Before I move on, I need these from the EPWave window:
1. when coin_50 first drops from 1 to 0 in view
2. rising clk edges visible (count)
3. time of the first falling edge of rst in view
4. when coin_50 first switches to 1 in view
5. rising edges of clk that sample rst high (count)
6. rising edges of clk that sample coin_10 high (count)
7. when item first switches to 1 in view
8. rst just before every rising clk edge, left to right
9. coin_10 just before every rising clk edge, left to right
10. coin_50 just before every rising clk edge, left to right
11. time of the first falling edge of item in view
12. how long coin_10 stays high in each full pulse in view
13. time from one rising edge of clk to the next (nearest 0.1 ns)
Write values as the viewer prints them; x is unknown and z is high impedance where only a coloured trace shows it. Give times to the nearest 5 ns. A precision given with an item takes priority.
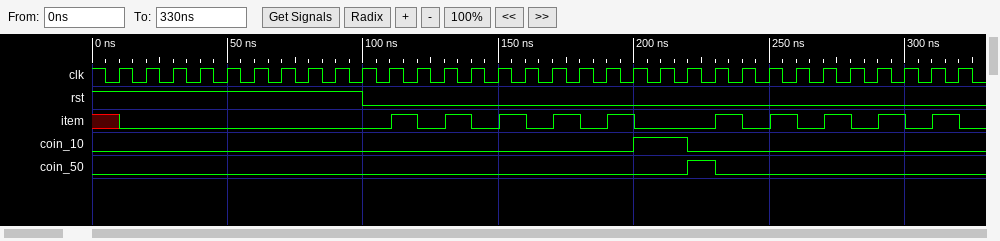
230 ns
32
100 ns
220 ns
10
2
110 ns
1 1 1 1 1 1 1 1 1 1 0 0 0 0 0 0 0 0 0 0 0 0 0 0 0 0 0 0 0 0 0 0
0 0 0 0 0 0 0 0 0 0 0 0 0 0 0 0 0 0 0 0 1 1 0 0 0 0 0 0 0 0 0 0
0 0 0 0 0 0 0 0 0 0 0 0 0 0 0 0 0 0 0 0 0 0 1 0 0 0 0 0 0 0 0 0
120 ns
20 ns
10 ns
